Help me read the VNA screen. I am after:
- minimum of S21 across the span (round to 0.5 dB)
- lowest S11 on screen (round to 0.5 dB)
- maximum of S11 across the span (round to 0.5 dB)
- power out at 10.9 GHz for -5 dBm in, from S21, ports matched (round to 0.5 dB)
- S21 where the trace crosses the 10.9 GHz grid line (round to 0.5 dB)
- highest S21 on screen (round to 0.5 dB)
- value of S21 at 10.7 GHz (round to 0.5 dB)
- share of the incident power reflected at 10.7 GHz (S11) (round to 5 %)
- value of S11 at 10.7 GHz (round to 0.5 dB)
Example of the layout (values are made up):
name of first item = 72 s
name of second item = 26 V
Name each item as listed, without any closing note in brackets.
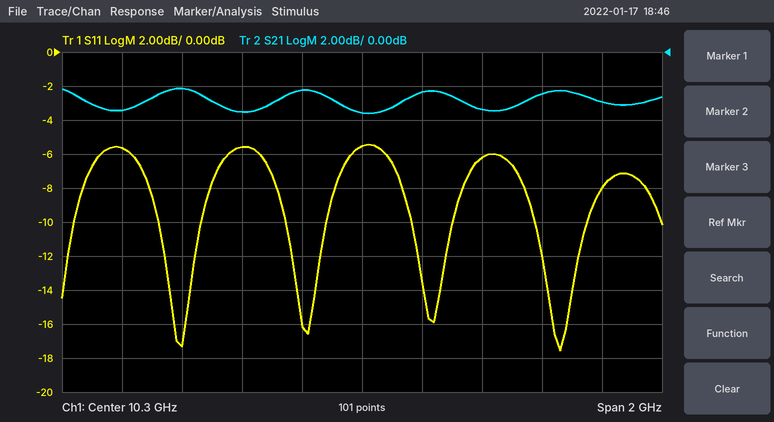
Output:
minimum of S21 across the span = -3.5 dB
lowest S11 on screen = -17.5 dB
maximum of S11 across the span = -5.5 dB
power out at 10.9 GHz for -5 dBm in, from S21, ports matched = -7.5 dBm
S21 where the trace crosses the 10.9 GHz grid line = -2.5 dB
highest S21 on screen = -2.0 dB
value of S21 at 10.7 GHz = -3.5 dB
share of the incident power reflected at 10.7 GHz (S11) = 25 %
value of S11 at 10.7 GHz = -6.0 dB
